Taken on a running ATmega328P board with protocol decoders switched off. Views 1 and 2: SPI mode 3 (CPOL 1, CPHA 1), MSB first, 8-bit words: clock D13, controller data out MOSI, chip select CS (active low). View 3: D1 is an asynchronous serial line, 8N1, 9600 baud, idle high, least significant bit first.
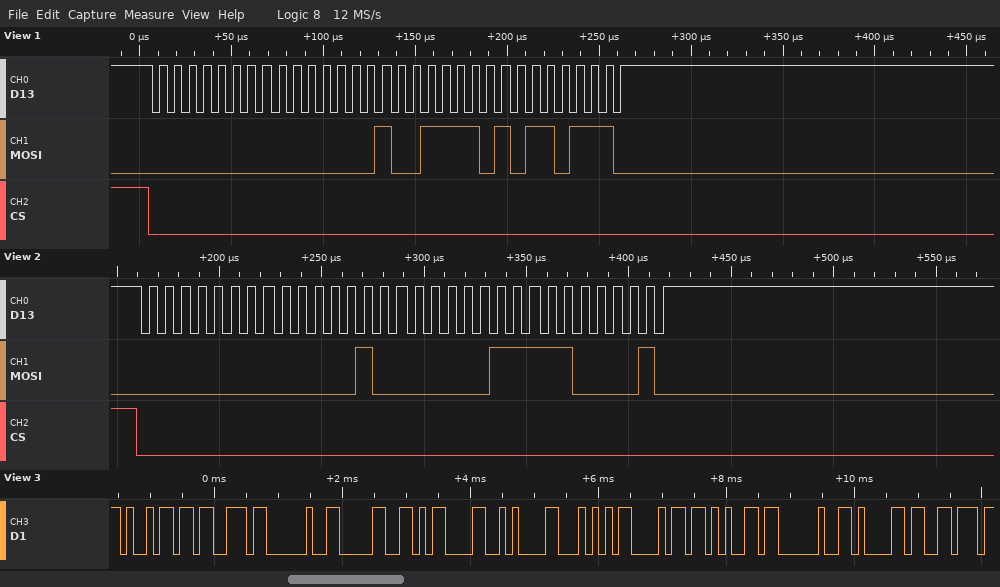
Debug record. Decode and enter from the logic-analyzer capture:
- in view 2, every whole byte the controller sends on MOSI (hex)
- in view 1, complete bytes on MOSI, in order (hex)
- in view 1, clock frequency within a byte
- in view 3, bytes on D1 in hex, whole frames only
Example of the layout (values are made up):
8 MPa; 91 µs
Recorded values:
00 04 07 C2; 00 01 3D 6E; 125 kHz; 0x69 0x73 0x20 0x30 0x0D 0x0A 0x54 0x68 0x65 0x20 0x61 0x76
